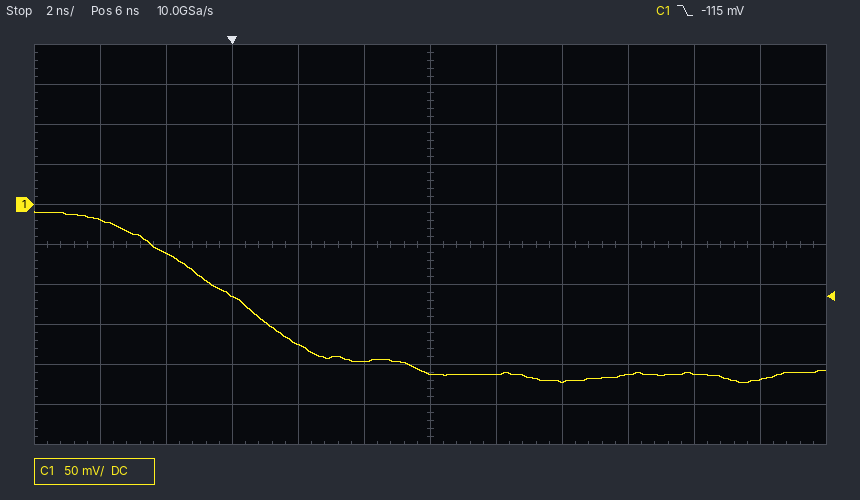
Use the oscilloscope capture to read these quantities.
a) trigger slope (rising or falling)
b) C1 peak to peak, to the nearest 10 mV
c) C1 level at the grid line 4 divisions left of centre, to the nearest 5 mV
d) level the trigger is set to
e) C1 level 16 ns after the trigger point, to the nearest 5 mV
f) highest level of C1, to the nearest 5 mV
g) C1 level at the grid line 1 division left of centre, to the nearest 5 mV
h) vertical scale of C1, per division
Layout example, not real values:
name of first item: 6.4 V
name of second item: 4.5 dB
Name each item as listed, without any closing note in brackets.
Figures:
trigger slope: falling
C1 peak to peak, to the nearest 10 mV: 210 mV
C1 level at the grid line 4 divisions left of centre, to the nearest 5 mV: -60 mV
level the trigger is set to: -115 mV
C1 level 16 ns after the trigger point, to the nearest 5 mV: -220 mV
highest level of C1, to the nearest 5 mV: -10 mV
C1 level at the grid line 1 division left of centre, to the nearest 5 mV: -195 mV
vertical scale of C1, per division: 50 mV
